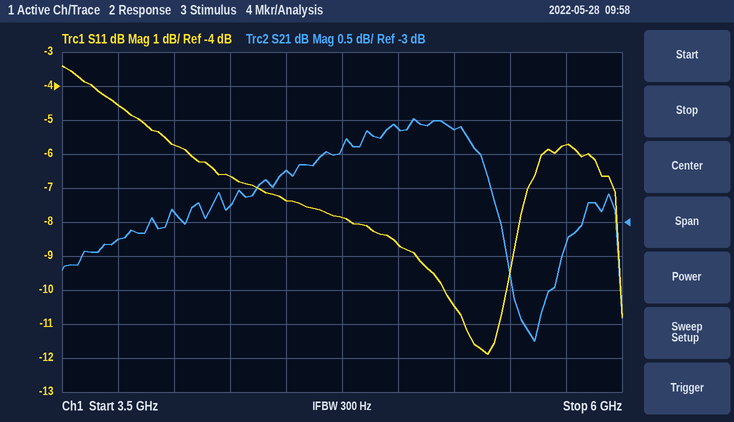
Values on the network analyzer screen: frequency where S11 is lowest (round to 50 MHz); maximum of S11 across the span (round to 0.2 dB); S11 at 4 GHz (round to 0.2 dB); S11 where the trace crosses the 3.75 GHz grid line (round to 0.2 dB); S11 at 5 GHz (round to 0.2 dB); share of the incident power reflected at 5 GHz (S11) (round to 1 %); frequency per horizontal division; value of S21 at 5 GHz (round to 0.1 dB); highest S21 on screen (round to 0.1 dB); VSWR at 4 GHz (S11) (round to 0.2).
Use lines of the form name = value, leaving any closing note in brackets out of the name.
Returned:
frequency where S11 is lowest = 5.40 GHz
maximum of S11 across the span = -3.4 dB
S11 at 4 GHz = -5.8 dB
S11 where the trace crosses the 3.75 GHz grid line = -4.6 dB
S11 at 5 GHz = -8.6 dB
share of the incident power reflected at 5 GHz (S11) = 14 %
frequency per horizontal division = 250 MHz
value of S21 at 5 GHz = -1.6 dB
highest S21 on screen = -1.5 dB
VSWR at 4 GHz (S11) = 3.2
